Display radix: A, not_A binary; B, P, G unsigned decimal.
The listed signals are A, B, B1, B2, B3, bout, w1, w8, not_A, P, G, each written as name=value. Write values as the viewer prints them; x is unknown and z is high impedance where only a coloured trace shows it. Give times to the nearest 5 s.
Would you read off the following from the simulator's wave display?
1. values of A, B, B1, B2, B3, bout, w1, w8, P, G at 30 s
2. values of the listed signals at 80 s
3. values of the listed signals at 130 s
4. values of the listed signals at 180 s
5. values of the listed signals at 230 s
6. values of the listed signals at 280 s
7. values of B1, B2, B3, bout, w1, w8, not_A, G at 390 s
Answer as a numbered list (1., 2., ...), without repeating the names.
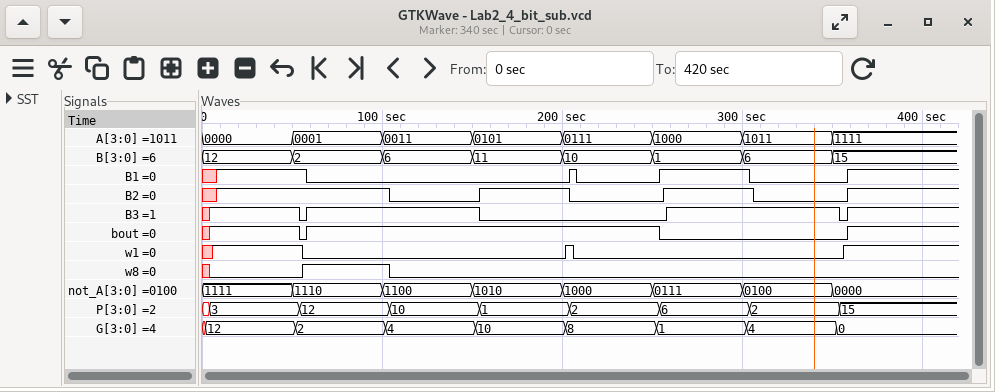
1. A=0000, B=12, B1=1, B2=1, B3=1, bout=1, w1=1, w8=0, P=3, G=12
2. A=0001, B=2, B1=0, B2=1, B3=1, bout=1, w1=0, w8=1, not_A=1110, P=12, G=2
3. A=0011, B=6, B1=0, B2=0, B3=1, bout=1, w1=0, w8=0, not_A=1100, P=10, G=4
4. A=0101, B=11, B1=0, B2=1, B3=0, bout=1, w1=0, w8=0, not_A=1010, P=1, G=10
5. A=0111, B=10, B1=0, B2=0, B3=0, bout=1, w1=0, w8=0, not_A=1000, P=2, G=8
6. A=1000, B=1, B1=1, B2=1, B3=1, bout=0, w1=0, w8=0, not_A=0111, P=6, G=1
7. B1=1, B2=1, B3=1, bout=1, w1=1, w8=0, not_A=0000, G=0
